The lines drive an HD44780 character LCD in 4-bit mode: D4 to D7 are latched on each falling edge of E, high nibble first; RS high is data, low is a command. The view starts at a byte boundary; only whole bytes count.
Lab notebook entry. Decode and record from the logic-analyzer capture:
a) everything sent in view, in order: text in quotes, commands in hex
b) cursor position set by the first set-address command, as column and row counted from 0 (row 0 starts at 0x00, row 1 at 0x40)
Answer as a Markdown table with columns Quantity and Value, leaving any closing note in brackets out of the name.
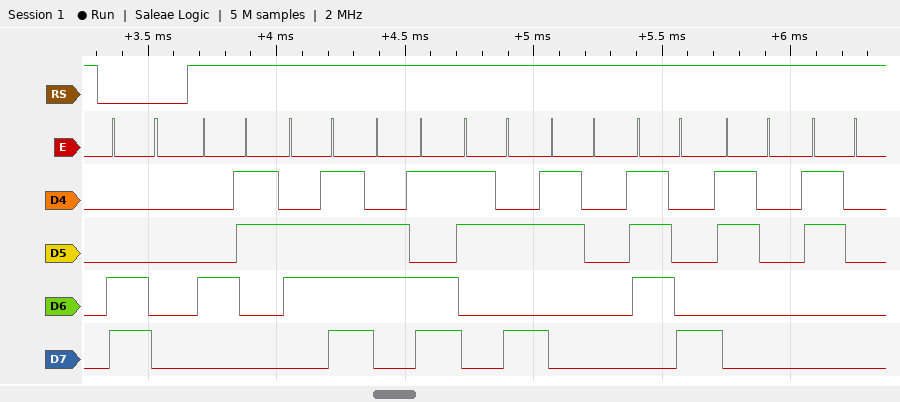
| Quantity | Value |
|---|---|
| everything sent in view, in order: text in quotes, commands in hex | 0xC0 "Com:0x00" |
| cursor position set by the first set-address command, as column and row counted from 0 | column 0, row 1 |
